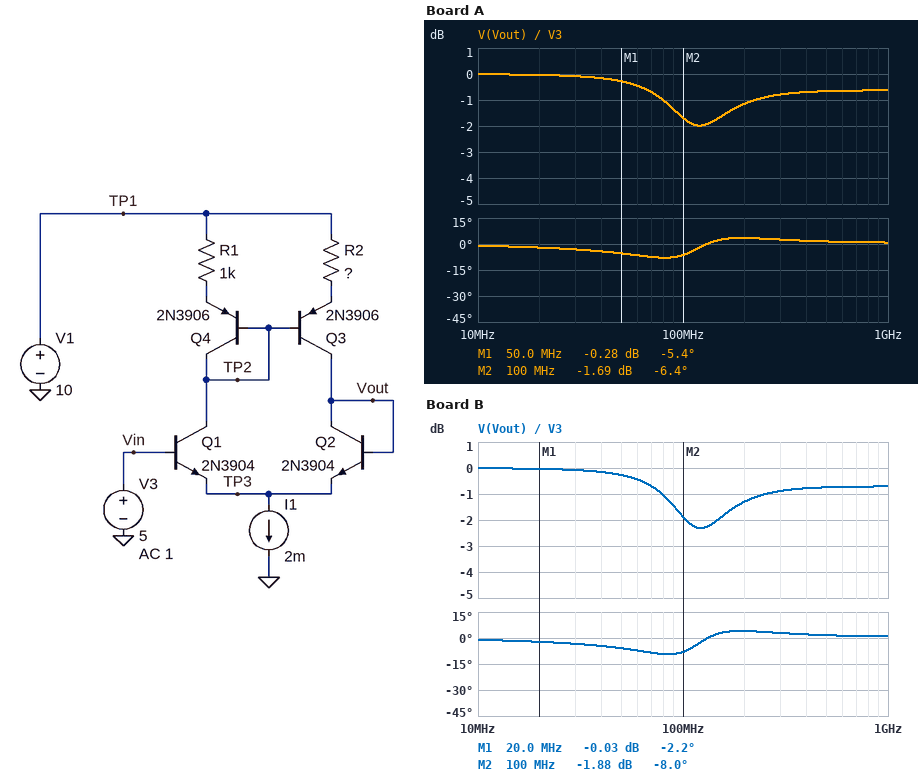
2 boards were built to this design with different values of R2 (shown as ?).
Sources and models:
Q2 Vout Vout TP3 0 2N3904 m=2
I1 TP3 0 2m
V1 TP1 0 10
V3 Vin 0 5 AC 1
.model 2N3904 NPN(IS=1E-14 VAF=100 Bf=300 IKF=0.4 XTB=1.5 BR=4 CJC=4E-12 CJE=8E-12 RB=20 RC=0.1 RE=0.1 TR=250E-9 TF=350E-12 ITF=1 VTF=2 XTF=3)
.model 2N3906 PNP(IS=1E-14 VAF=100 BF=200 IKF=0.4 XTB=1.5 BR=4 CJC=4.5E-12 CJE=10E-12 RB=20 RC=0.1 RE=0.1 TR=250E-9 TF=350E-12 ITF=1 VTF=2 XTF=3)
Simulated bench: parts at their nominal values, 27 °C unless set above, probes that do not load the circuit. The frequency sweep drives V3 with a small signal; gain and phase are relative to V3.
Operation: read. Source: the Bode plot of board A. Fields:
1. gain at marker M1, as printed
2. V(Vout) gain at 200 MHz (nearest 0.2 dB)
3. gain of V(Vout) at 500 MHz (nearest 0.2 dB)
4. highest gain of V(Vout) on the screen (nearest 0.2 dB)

-0.28 dB
-1.2 dB
-0.6 dB
0 dB
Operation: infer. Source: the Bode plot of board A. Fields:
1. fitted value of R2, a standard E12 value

470 Ω
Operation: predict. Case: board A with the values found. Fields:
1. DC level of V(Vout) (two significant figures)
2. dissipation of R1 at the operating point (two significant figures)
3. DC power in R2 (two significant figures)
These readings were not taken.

5.0 V
420 µW
850 µW
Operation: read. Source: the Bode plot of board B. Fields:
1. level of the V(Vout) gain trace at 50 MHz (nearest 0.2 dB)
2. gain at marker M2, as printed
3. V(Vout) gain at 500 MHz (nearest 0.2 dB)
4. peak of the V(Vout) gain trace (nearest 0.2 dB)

-0.2 dB
-1.88 dB
-0.8 dB
0 dB
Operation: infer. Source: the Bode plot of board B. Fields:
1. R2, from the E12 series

390 Ω
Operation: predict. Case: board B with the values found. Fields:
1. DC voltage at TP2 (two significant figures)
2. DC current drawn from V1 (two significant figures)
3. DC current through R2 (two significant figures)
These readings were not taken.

8.8 V
2.0 mA
1.4 mA
